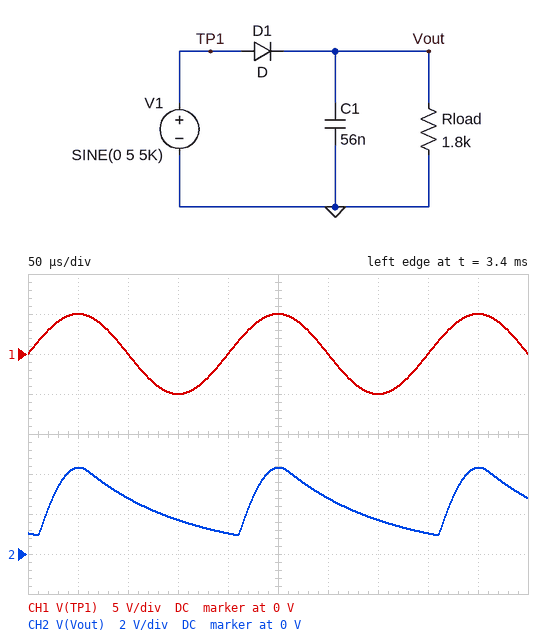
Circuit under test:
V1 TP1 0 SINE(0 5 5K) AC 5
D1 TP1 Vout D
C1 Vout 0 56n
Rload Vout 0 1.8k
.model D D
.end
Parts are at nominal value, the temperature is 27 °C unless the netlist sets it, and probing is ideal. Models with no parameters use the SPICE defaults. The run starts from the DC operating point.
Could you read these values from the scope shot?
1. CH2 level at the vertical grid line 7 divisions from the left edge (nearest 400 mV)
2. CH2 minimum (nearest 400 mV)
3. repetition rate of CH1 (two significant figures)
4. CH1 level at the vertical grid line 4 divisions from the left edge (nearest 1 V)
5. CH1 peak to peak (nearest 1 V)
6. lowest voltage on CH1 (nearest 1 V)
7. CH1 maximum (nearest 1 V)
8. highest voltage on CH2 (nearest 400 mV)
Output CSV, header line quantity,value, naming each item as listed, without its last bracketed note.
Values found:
quantity,value
CH2 level at the vertical grid line 7 divisions from the left edge,1.6 V
CH2 minimum,800 mV
repetition rate of CH1,5.0 kHz
CH1 level at the vertical grid line 4 divisions from the left edge,0 V
CH1 peak to peak,10 V
lowest voltage on CH1,-5 V
CH1 maximum,5 V
highest voltage on CH2,4.4 V
